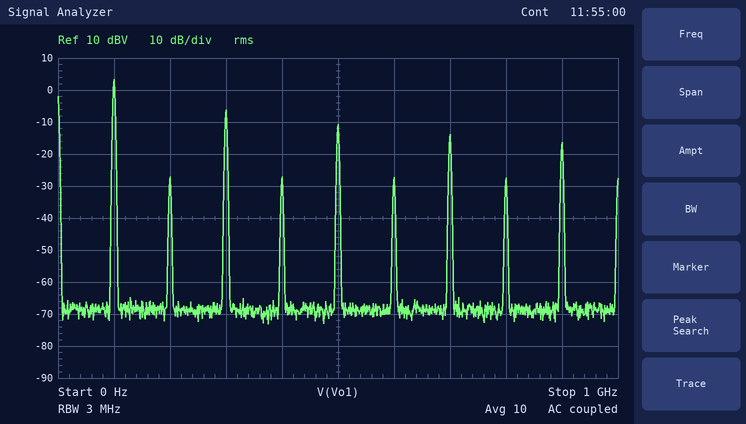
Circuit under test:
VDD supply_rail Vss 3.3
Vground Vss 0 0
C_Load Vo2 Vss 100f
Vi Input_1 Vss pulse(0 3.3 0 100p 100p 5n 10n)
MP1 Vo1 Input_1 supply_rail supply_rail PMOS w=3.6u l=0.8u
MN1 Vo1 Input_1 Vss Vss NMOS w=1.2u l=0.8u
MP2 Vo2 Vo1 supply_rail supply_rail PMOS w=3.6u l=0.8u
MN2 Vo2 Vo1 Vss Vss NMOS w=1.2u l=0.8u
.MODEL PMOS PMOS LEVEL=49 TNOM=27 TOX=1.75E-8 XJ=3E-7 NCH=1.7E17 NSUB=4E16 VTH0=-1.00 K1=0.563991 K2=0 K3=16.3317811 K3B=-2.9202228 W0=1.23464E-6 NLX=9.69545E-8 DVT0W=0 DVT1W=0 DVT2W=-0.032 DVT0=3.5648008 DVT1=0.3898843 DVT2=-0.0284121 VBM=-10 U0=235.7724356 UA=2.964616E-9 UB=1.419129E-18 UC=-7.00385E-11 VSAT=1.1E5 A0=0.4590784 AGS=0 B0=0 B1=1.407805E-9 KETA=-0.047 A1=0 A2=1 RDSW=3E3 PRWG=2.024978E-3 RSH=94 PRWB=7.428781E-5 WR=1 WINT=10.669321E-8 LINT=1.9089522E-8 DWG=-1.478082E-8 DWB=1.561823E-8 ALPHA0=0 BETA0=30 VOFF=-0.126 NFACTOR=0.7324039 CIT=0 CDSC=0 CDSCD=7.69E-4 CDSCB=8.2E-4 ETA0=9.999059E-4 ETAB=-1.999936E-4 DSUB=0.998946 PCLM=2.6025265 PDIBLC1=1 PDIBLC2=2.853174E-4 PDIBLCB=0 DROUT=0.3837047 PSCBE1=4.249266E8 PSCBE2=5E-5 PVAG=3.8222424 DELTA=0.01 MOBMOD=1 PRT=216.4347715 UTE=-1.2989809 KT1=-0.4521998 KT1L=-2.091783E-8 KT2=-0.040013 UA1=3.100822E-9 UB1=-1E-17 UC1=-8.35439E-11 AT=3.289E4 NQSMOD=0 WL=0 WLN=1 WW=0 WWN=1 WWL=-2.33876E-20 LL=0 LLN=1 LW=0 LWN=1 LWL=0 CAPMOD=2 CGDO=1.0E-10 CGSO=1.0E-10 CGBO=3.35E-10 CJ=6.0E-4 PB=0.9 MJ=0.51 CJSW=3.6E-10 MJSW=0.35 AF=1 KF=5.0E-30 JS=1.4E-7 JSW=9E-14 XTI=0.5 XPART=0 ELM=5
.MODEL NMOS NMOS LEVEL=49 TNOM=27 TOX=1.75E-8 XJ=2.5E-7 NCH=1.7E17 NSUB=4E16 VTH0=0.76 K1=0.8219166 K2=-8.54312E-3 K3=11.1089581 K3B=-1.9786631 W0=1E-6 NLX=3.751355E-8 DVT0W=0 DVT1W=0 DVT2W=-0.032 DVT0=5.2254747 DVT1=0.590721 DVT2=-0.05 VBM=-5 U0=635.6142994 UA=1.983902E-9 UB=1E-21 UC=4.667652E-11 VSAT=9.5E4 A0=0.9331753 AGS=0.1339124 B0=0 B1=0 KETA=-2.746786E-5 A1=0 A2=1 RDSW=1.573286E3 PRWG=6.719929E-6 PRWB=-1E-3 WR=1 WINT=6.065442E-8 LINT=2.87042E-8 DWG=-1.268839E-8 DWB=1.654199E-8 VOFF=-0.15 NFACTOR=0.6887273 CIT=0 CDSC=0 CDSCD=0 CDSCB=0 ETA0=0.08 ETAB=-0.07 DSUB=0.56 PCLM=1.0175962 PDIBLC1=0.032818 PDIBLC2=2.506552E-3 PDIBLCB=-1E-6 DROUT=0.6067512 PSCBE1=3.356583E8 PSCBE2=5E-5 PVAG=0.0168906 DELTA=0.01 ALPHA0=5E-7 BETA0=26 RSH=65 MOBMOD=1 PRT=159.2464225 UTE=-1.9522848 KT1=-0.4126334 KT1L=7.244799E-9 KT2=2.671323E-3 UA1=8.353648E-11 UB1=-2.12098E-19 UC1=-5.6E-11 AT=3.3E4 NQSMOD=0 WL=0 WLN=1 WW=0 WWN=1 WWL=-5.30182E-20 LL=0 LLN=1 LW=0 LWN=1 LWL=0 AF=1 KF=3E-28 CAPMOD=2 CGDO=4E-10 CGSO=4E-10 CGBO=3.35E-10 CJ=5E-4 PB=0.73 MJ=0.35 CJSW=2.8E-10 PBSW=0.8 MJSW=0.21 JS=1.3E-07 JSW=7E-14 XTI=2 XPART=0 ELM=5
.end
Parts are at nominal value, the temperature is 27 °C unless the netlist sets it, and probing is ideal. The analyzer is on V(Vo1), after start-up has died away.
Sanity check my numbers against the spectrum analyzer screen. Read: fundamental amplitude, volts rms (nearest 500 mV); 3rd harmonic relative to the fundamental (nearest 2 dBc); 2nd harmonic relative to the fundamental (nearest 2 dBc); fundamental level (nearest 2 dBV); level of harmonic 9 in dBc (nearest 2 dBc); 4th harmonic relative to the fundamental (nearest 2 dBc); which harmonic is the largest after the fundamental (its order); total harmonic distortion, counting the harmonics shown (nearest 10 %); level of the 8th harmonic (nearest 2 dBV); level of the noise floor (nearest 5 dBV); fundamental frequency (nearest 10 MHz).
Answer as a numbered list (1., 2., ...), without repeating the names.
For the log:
1. 1.5 V
2. -10 dBc
3. -30 dBc
4. 4 dBV
5. -20 dBc
6. -30 dBc
7. 3
8. 40 %
9. -28 dBV
10. -70 dBV
11. 100 MHz
